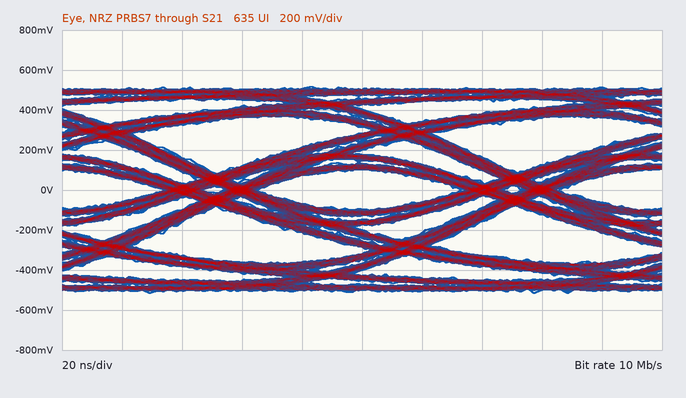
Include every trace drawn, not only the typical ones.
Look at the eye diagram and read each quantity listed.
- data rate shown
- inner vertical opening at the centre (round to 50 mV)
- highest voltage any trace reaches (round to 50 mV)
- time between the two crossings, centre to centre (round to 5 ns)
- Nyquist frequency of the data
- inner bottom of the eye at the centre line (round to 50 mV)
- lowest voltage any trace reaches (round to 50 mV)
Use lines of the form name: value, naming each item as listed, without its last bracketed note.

data rate shown: 10 Mb/s
inner vertical opening at the centre: 200 mV
highest voltage any trace reaches: 500 mV
time between the two crossings, centre to centre: 100 ns
Nyquist frequency of the data: 5 MHz
inner bottom of the eye at the centre line: -100 mV
lowest voltage any trace reaches: -500 mV
